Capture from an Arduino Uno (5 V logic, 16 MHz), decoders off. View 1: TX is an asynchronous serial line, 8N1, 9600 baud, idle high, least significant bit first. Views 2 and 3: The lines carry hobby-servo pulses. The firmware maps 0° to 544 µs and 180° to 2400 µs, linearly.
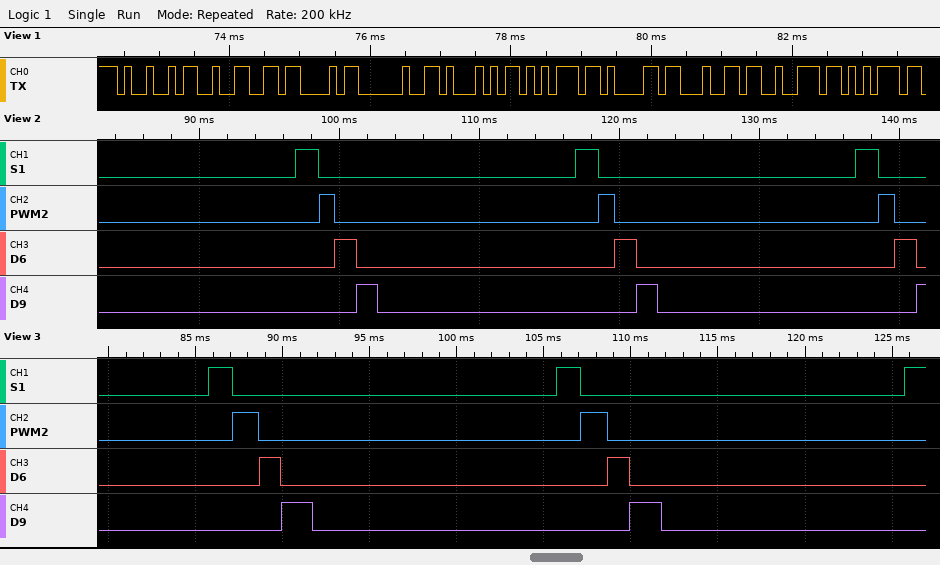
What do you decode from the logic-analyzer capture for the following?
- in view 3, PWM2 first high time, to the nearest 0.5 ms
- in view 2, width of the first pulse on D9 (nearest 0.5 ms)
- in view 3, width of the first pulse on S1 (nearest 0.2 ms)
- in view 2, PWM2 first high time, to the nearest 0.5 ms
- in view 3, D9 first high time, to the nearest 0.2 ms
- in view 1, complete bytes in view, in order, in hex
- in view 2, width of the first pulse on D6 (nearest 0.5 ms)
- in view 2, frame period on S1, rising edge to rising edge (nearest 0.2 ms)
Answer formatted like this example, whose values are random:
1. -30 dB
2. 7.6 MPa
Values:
1. 1.5 ms
2. 1.5 ms
3. 1.4 ms
4. 1.0 ms
5. 1.8 ms
6. 49 32 43 20 51 75 61 64 72 75
7. 1.5 ms
8. 20.0 ms
